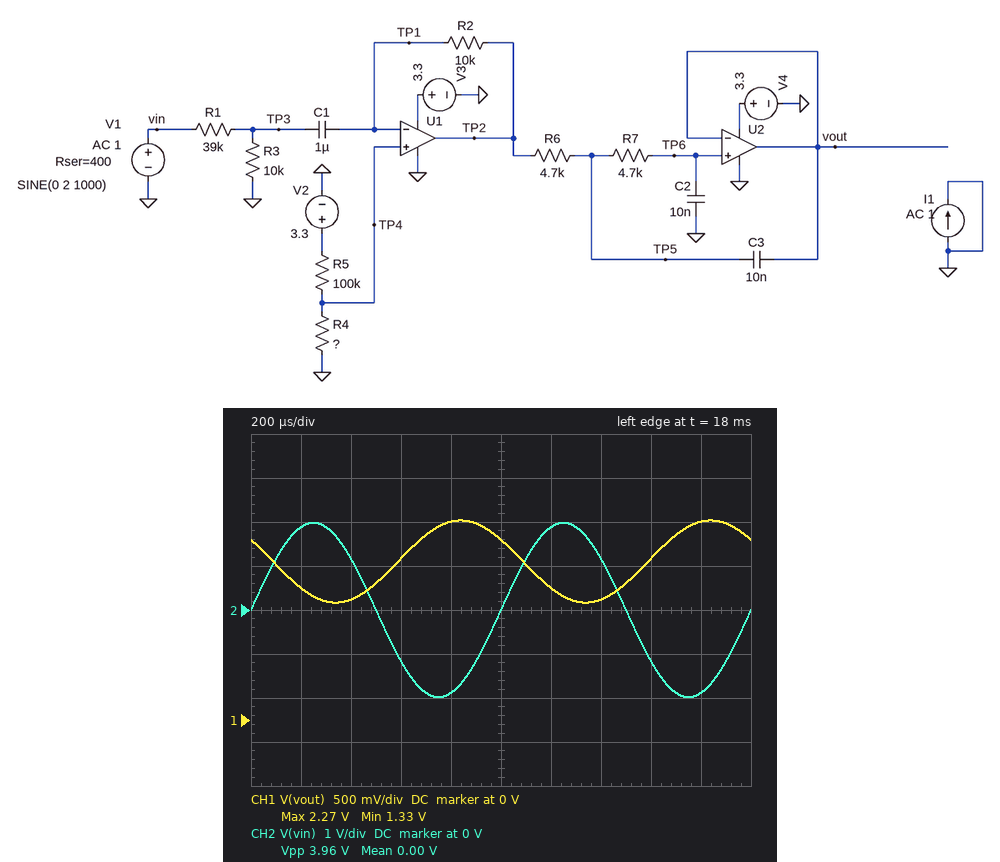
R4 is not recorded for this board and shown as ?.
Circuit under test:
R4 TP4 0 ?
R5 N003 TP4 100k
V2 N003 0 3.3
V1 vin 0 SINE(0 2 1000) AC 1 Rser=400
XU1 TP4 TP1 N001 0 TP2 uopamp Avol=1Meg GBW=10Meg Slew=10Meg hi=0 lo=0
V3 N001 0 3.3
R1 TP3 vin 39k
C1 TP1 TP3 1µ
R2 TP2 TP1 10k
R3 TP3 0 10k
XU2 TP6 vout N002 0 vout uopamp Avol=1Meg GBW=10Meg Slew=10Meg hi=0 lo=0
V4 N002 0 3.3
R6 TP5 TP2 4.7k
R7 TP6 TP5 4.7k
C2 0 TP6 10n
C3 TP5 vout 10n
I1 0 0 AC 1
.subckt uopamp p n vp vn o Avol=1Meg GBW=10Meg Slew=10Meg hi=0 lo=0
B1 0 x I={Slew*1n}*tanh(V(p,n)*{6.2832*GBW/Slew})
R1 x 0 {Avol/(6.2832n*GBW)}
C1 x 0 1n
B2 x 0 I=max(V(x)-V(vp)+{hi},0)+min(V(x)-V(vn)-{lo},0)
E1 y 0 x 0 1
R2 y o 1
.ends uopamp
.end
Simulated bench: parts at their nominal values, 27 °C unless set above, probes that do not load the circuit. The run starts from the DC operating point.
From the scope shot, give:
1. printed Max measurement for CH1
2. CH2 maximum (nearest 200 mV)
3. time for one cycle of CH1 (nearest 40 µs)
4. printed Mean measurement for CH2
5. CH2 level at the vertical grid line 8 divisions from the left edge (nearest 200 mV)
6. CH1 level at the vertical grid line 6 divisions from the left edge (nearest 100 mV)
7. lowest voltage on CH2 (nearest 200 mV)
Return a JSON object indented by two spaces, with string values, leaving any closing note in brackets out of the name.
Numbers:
{
  "printed Max measurement for CH1": "2.27 V",
  "CH2 maximum": "2.0 V",
  "time for one cycle of CH1": "1.00 ms",
  "printed Mean measurement for CH2": "0.00 V",
  "CH2 level at the vertical grid line 8 divisions from the left edge": "-1.2 V",
  "CH1 level at the vertical grid line 6 divisions from the left edge": "1.5 V",
  "lowest voltage on CH2": "-2.0 V"
}
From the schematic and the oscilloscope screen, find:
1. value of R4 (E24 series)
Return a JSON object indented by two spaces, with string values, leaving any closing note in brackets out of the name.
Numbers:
{
  "value of R4": "120 kΩ"
}
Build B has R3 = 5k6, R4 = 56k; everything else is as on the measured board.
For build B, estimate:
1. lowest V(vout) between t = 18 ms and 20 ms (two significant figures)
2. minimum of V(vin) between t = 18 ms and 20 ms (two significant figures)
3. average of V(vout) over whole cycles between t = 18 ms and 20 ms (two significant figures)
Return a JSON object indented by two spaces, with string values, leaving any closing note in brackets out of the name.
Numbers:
{
  "lowest V(vout) between t = 18 ms and 20 ms": "720 mV",
  "minimum of V(vin) between t = 18 ms and 20 ms": "-2.0 V",
  "average of V(vout) over whole cycles between t = 18 ms and 20 ms": "1.2 V"
}
